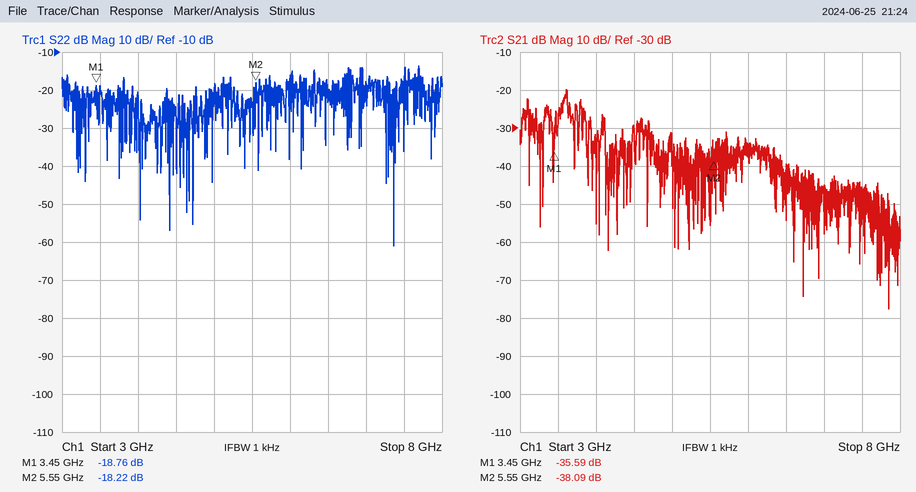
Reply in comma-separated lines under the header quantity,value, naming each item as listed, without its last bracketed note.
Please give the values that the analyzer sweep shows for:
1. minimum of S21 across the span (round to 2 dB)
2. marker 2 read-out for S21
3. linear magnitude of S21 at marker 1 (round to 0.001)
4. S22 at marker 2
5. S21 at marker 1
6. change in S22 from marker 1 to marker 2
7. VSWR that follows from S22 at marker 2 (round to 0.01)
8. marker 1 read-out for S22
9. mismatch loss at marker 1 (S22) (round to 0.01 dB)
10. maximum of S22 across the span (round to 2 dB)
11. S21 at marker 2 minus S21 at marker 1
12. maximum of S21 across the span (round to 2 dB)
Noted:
quantity,value
minimum of S21 across the span,-78 dB
marker 2 read-out for S21,-38.09 dB
linear magnitude of S21 at marker 1,0.017
S22 at marker 2,-18.22 dB
S21 at marker 1,-35.59 dB
change in S22 from marker 1 to marker 2,0.54 dB
VSWR that follows from S22 at marker 2,1.28
marker 1 read-out for S22,-18.76 dB
mismatch loss at marker 1 (S22),0.06 dB
maximum of S22 across the span,-14 dB
S21 at marker 2 minus S21 at marker 1,-2.50 dB
maximum of S21 across the span,-20 dB
